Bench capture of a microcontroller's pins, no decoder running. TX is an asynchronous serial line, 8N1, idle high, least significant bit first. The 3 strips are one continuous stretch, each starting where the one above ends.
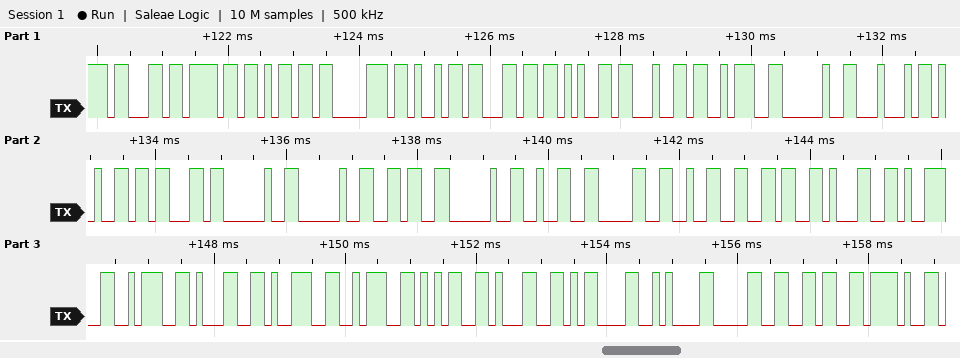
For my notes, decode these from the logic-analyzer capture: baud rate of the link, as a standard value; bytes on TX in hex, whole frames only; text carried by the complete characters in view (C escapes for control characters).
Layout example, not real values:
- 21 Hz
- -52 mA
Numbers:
- 9600 baud
- 63 6F 6D 70 69 6C 65 64 3A 20 44 65 63 20 20 36 20 32 30 32 36 31 39 3A 31 39 3A 35 31 0D 0A 30 36 2F
- "compiled: Dec  6 202619:19:51\r\n06/"
